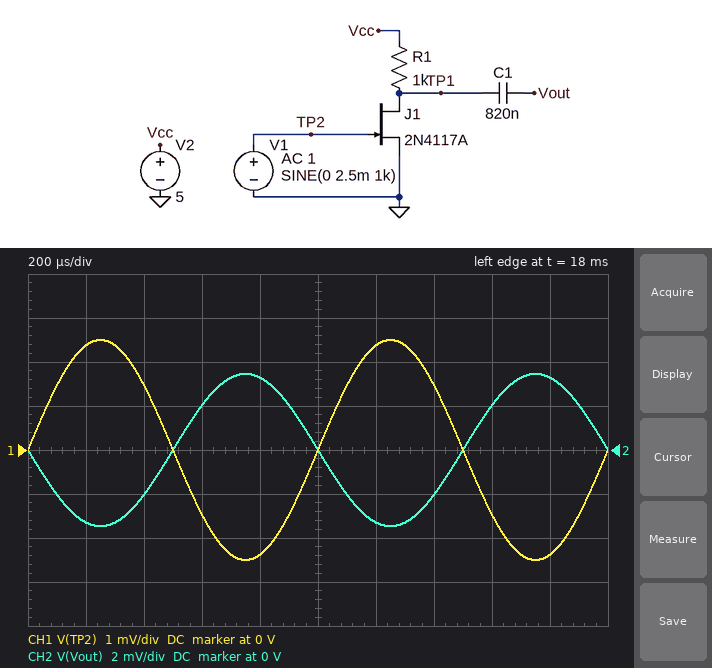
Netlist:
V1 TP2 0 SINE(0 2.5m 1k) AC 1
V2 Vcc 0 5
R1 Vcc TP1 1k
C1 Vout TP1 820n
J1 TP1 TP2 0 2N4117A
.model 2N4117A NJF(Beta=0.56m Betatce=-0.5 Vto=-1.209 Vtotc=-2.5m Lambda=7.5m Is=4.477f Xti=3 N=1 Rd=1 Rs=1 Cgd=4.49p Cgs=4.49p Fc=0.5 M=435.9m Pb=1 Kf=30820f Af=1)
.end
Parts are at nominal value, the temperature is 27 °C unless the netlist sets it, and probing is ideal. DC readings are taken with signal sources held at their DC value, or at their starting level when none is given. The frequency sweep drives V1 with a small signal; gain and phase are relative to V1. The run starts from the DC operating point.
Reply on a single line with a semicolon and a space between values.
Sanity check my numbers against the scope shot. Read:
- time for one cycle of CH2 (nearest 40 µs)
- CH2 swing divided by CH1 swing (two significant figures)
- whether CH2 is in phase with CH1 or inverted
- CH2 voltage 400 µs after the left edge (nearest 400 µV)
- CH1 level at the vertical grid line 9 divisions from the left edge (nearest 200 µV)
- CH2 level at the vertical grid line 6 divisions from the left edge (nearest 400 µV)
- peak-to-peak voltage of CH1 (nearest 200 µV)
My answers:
1.00 ms; 1.4; inverted; -2.0 mV; -2.4 mV; -3.2 mV; 5.0 mV
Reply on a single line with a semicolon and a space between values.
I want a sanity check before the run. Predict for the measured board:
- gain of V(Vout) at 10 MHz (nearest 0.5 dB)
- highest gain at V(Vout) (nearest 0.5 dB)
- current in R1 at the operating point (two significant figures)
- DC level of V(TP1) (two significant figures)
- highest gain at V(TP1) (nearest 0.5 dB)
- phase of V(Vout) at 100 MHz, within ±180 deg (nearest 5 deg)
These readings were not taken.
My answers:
3.0 dB; 3.0 dB; 840 µA; 4.2 V; 3.0 dB; 85 deg
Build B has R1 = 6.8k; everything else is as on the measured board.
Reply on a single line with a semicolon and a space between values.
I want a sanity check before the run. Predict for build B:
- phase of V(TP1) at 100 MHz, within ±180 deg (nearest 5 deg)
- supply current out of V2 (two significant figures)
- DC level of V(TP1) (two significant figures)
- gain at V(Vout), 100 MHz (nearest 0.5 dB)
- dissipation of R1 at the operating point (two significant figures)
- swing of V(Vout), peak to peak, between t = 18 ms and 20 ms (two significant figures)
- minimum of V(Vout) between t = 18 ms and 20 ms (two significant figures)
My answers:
40 deg; 640 µA; 640 mV; 0 dB; 2.8 mW; 4.6 mV; -2.3 mV
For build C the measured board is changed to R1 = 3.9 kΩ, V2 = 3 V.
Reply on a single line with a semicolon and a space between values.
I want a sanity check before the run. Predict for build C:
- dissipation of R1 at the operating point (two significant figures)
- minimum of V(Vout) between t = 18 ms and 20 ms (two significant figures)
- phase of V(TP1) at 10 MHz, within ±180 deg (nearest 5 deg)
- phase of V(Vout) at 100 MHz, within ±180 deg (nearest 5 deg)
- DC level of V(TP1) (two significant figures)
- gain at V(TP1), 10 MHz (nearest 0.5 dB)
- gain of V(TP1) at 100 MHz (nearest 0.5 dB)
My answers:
1.5 mW; -1.8 mV; 150 deg; 40 deg; 600 mV; -2.5 dB; -0.5 dB
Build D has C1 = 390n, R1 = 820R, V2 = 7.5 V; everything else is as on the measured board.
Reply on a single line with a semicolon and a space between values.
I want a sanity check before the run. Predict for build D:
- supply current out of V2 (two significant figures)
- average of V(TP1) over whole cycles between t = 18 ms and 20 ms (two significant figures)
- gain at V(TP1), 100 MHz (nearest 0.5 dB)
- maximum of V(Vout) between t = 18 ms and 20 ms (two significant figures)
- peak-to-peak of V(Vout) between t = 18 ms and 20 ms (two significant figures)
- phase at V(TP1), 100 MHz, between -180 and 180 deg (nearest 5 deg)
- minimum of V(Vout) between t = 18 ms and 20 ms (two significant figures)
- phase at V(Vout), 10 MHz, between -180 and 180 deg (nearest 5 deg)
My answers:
860 µA; 6.8 V; 1.0 dB; 2.9 mV; 5.8 mV; 105 deg; -2.9 mV; 170 deg
